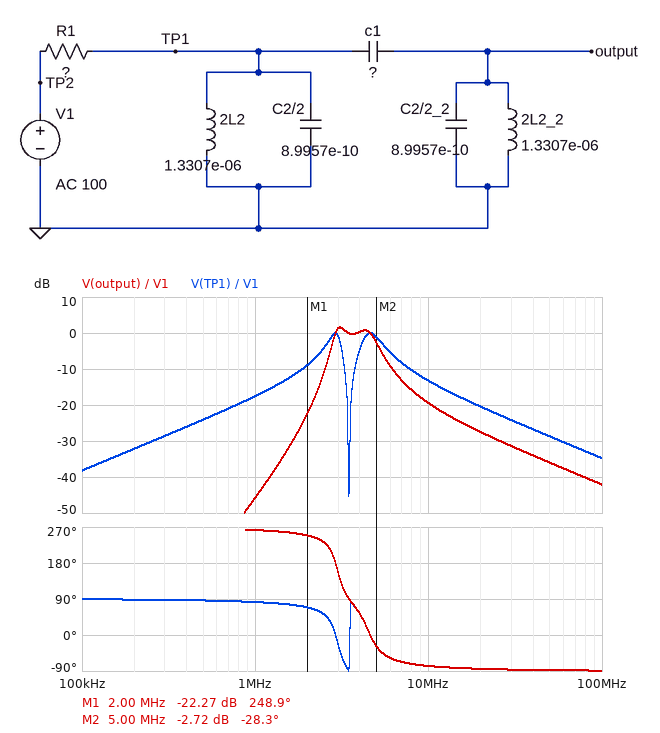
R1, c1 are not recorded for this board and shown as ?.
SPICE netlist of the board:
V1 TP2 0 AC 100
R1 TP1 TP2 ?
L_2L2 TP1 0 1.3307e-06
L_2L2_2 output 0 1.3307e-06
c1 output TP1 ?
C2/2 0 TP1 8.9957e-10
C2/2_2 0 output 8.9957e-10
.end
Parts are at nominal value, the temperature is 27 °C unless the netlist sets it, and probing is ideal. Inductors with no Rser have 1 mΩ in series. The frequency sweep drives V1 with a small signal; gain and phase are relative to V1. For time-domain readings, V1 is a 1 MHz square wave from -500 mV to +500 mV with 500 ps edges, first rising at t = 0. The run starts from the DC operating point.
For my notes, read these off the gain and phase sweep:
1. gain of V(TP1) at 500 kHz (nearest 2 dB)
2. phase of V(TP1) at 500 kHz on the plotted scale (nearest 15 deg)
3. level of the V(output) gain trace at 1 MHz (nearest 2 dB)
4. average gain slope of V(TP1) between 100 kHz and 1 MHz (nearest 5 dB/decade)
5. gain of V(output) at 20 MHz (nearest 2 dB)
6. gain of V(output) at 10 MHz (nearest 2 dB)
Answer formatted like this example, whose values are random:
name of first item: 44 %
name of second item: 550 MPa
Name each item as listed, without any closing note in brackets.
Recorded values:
gain of V(TP1) at 500 kHz: -24 dB
phase of V(TP1) at 500 kHz on the plotted scale: 90 deg
level of the V(output) gain trace at 1 MHz: -46 dB
average gain slope of V(TP1) between 100 kHz and 1 MHz: 20 dB/decade
gain of V(output) at 20 MHz: -28 dB
gain of V(output) at 10 MHz: -20 dB
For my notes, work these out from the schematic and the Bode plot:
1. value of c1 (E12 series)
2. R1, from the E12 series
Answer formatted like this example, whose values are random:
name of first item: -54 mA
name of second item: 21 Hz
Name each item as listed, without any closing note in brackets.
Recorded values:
value of c1: 680 pF
R1, from the E12 series: 68 Ω
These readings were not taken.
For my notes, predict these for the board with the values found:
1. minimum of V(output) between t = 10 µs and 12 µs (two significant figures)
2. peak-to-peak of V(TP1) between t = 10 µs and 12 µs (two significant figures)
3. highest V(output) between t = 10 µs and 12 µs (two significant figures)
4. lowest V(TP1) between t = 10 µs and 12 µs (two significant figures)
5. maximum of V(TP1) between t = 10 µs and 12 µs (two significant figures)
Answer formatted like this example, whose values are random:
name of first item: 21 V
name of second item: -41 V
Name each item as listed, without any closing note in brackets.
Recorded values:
minimum of V(output) between t = 10 µs and 12 µs: -330 mV
peak-to-peak of V(TP1) between t = 10 µs and 12 µs: 750 mV
highest V(output) between t = 10 µs and 12 µs: 330 mV
lowest V(TP1) between t = 10 µs and 12 µs: -380 mV
maximum of V(TP1) between t = 10 µs and 12 µs: 380 mV
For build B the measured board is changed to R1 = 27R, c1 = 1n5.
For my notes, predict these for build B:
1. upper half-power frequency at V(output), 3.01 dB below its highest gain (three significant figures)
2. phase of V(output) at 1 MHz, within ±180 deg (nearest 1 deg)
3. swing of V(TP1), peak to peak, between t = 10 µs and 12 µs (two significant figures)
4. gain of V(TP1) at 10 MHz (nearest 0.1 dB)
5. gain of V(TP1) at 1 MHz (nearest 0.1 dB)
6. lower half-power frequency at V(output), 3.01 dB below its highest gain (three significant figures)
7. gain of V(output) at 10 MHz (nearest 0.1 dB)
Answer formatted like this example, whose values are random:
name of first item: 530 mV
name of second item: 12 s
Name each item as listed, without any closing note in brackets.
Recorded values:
upper half-power frequency at V(output), 3.01 dB below its highest gain: 4.37 MHz
phase of V(output) at 1 MHz, within ±180 deg: -110 deg
swing of V(TP1), peak to peak, between t = 10 µs and 12 µs: 970 mV
gain of V(TP1) at 10 MHz: -7.1 dB
gain of V(TP1) at 1 MHz: -9.5 dB
lower half-power frequency at V(output), 3.01 dB below its highest gain: 2.23 MHz
gain of V(output) at 10 MHz: -10.4 dB
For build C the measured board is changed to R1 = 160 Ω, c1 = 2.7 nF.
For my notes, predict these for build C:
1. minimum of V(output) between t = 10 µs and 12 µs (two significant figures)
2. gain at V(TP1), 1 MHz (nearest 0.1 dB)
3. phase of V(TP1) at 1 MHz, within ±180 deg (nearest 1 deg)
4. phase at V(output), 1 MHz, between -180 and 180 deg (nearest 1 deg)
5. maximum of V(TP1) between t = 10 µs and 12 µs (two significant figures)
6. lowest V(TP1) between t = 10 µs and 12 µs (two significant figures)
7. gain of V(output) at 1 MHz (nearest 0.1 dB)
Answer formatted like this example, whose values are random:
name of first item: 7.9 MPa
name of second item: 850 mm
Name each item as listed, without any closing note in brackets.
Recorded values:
minimum of V(output) between t = 10 µs and 12 µs: -110 mV
gain at V(TP1), 1 MHz: -23.6 dB
phase of V(TP1) at 1 MHz, within ±180 deg: 86 deg
phase at V(output), 1 MHz, between -180 and 180 deg: -94 deg
maximum of V(TP1) between t = 10 µs and 12 µs: 130 mV
lowest V(TP1) between t = 10 µs and 12 µs: -130 mV
gain of V(output) at 1 MHz: -38.7 dB
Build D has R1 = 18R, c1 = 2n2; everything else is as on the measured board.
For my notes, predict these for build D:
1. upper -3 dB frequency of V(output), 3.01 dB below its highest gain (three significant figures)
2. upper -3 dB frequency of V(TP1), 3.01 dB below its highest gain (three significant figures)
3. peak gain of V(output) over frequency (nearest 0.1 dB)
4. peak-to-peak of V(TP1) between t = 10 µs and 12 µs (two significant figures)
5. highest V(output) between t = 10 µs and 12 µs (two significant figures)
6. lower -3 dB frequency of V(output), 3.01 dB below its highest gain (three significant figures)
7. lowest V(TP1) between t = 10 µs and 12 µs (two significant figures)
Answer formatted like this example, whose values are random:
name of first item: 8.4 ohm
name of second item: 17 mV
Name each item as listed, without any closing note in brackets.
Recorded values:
upper -3 dB frequency of V(output), 3.01 dB below its highest gain: 3.52 MHz
upper -3 dB frequency of V(TP1), 3.01 dB below its highest gain: 8.12 MHz
peak gain of V(output) over frequency: 4.6 dB
peak-to-peak of V(TP1) between t = 10 µs and 12 µs: 1.4 V
highest V(output) between t = 10 µs and 12 µs: 460 mV
lower -3 dB frequency of V(output), 3.01 dB below its highest gain: 1.97 MHz
lowest V(TP1) between t = 10 µs and 12 µs: -690 mV
